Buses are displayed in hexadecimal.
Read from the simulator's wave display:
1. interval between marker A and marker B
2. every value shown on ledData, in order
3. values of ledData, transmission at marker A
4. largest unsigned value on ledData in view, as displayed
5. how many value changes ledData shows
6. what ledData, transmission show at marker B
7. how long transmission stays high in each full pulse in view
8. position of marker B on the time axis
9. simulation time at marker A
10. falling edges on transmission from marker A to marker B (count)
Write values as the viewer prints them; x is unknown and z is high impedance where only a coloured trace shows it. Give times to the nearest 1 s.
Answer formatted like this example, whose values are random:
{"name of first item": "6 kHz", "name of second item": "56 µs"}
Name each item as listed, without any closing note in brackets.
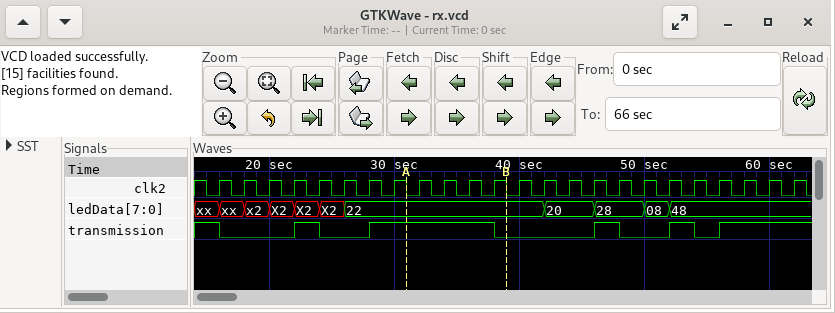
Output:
{"interval between marker A and marker B": "8 s", "every value shown on ledData, in order": "xx, xx, x2, X2, X2, X2, 22, 20, 28, 08, 48", "values of ledData, transmission at marker A": "ledData=22, transmission=1", "largest unsigned value on ledData in view, as displayed": "48", "how many value changes ledData shows": "10", "what ledData, transmission show at marker B": "ledData=22, transmission=0", "how long transmission stays high in each full pulse in view": "2 s, 10 s, 2 s, 2 s", "position of marker B on the time axis": "39 s", "simulation time at marker A": "31 s", "falling edges on transmission from marker A to marker B": "1"}
